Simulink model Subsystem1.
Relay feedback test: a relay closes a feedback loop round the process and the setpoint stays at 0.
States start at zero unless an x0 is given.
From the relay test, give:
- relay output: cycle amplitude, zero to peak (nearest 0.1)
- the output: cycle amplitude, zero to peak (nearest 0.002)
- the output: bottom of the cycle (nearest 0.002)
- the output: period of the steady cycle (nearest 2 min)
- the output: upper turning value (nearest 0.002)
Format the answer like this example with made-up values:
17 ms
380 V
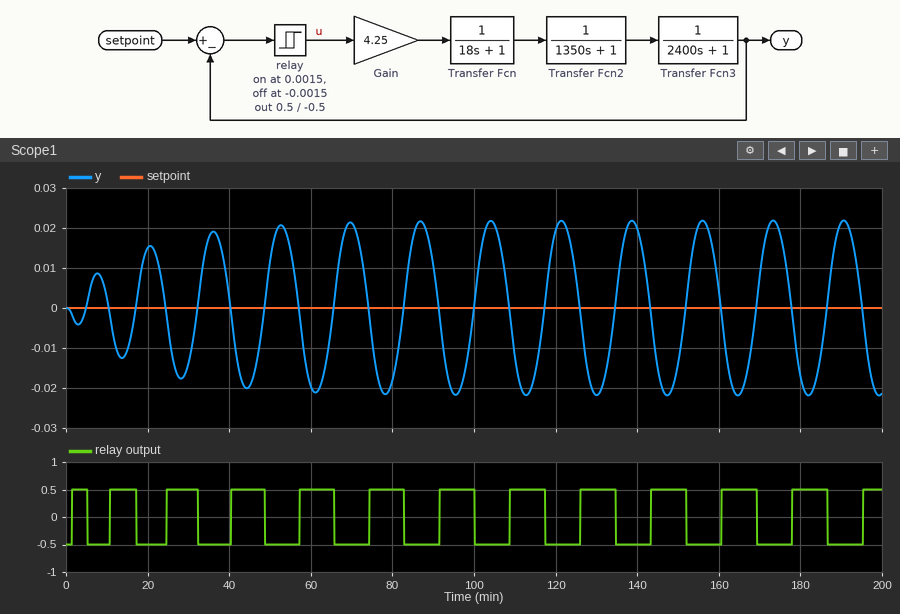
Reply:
0.5
0.022
-0.022
18 min
0.022
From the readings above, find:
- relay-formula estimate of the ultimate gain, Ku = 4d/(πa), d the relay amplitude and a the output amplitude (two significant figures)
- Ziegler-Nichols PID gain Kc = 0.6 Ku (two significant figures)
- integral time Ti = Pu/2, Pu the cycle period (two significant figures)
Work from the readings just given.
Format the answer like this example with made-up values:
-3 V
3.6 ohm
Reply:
29
17
9.0 min
